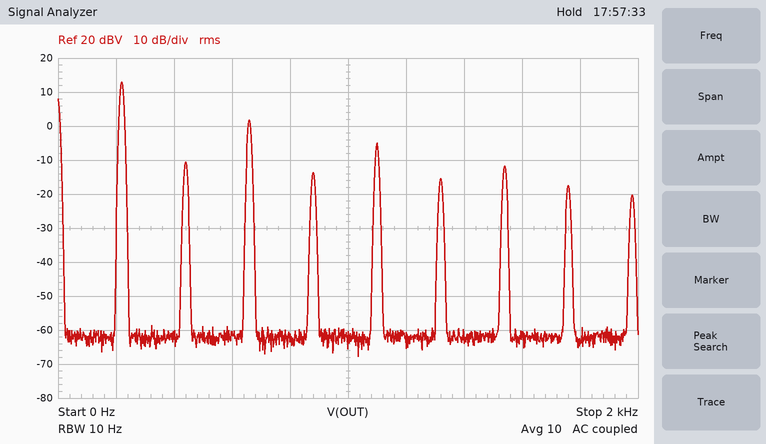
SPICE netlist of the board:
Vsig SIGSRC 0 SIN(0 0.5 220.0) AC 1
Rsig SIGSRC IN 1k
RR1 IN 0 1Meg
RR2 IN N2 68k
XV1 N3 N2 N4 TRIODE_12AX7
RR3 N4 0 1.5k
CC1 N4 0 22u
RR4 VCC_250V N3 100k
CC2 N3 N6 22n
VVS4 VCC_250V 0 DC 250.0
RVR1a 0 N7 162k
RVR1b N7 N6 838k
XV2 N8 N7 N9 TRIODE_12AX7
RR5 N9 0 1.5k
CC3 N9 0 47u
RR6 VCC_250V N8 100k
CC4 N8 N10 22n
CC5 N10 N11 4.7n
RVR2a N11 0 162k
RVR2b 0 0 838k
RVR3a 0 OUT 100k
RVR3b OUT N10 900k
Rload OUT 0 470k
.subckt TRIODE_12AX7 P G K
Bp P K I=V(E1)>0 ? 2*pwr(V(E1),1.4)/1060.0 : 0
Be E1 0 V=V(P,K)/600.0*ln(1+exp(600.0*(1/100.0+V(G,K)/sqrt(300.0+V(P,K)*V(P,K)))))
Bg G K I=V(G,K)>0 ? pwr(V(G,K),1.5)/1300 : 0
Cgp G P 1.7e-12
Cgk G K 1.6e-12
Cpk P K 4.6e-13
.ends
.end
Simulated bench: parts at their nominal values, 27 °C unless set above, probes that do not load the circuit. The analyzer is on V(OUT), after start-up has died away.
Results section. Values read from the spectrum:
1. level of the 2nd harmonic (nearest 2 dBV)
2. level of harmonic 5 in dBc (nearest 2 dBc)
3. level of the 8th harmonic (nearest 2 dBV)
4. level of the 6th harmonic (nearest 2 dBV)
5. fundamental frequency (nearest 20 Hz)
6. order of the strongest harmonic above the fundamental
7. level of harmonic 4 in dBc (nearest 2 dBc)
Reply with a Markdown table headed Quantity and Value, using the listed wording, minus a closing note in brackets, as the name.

| Quantity | Value |
|---|---|
| level of the 2nd harmonic | -10 dBV |
| level of harmonic 5 in dBc | -18 dBc |
| level of the 8th harmonic | -18 dBV |
| level of the 6th harmonic | -16 dBV |
| fundamental frequency | 220 Hz |
| order of the strongest harmonic above the fundamental | 3 |
| level of harmonic 4 in dBc | -26 dBc |
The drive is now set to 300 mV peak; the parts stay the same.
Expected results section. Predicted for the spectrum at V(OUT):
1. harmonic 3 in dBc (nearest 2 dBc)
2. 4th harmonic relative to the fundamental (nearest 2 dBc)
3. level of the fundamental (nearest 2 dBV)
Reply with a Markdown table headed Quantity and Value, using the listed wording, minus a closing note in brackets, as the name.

| Quantity | Value |
|---|---|
| harmonic 3 in dBc | -14 dBc |
| 4th harmonic relative to the fundamental | -26 dBc |
| level of the fundamental | 12 dBV |
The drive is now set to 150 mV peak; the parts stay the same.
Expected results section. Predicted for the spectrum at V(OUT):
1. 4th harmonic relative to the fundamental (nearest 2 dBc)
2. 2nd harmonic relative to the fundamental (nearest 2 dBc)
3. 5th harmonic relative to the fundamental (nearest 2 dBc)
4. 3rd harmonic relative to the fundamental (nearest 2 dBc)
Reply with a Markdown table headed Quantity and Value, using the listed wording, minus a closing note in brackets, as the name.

| Quantity | Value |
|---|---|
| 4th harmonic relative to the fundamental | -36 dBc |
| 2nd harmonic relative to the fundamental | -20 dBc |
| 5th harmonic relative to the fundamental | -38 dBc |
| 3rd harmonic relative to the fundamental | -28 dBc |
